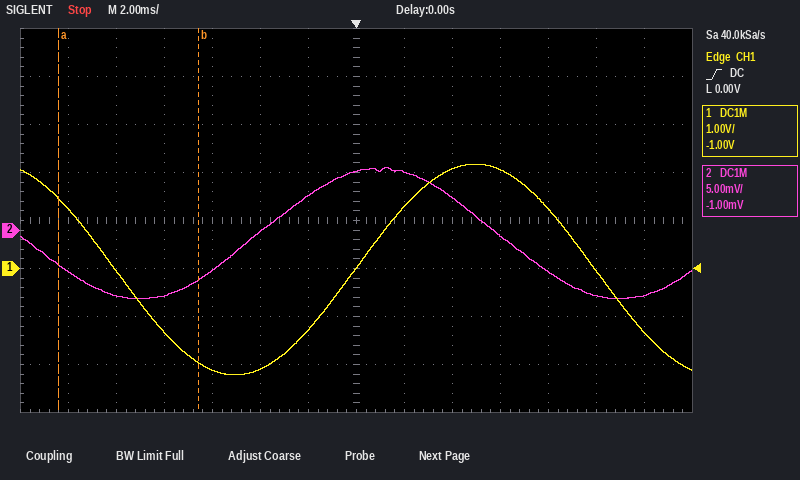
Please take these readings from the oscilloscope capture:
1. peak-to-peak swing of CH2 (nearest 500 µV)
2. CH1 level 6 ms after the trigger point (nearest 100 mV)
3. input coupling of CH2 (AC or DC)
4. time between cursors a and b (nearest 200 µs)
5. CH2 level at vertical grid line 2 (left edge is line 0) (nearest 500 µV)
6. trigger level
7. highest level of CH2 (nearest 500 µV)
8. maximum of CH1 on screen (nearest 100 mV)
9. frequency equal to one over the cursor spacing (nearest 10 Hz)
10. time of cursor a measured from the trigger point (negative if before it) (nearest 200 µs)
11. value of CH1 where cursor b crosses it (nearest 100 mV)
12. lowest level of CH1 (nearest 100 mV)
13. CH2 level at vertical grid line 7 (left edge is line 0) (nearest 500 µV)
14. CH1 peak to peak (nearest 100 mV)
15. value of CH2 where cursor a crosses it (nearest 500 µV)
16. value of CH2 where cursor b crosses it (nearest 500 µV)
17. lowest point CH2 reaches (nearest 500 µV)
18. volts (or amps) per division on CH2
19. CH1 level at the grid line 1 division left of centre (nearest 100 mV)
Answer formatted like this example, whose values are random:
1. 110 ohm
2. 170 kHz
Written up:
1. 13.5 mV
2. 2.1 V
3. DC
4. 5.8 ms
5. -7.0 mV
6. 0.00 V
7. 6.5 mV
8. 2.2 V
9. 170 Hz
10. -12.4 ms
11. -2.0 V
12. -2.2 V
13. 6.0 mV
14. 4.4 V
15. -3.5 mV
16. -5.0 mV
17. -7.0 mV
18. 5 mV
19. -1.3 V
